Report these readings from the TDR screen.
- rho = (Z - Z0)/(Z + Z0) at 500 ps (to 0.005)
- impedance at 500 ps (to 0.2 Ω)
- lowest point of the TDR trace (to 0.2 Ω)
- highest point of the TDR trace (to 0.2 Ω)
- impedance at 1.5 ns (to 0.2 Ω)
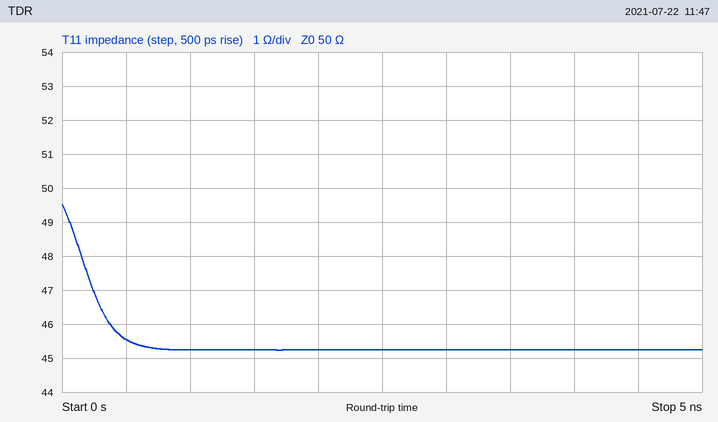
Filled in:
-0.045
45.6 Ω
45.2 Ω
49.6 Ω
45.2 Ω
